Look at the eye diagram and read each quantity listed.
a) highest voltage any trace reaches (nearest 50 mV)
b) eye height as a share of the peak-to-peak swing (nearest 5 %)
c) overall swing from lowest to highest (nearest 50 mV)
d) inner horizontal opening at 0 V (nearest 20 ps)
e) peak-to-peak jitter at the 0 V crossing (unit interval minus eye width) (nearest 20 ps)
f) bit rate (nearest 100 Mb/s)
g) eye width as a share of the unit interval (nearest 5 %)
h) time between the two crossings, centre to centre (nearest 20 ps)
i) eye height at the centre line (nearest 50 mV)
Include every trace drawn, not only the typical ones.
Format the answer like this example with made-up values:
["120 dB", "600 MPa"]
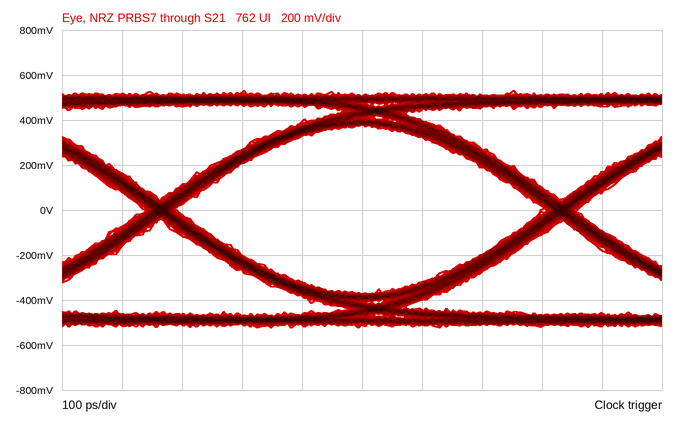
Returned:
["550 mV", "70 %", "1.05 V", "600 ps", "60 ps", "1.5 Gb/s", "90 %", "660 ps", "750 mV"]
